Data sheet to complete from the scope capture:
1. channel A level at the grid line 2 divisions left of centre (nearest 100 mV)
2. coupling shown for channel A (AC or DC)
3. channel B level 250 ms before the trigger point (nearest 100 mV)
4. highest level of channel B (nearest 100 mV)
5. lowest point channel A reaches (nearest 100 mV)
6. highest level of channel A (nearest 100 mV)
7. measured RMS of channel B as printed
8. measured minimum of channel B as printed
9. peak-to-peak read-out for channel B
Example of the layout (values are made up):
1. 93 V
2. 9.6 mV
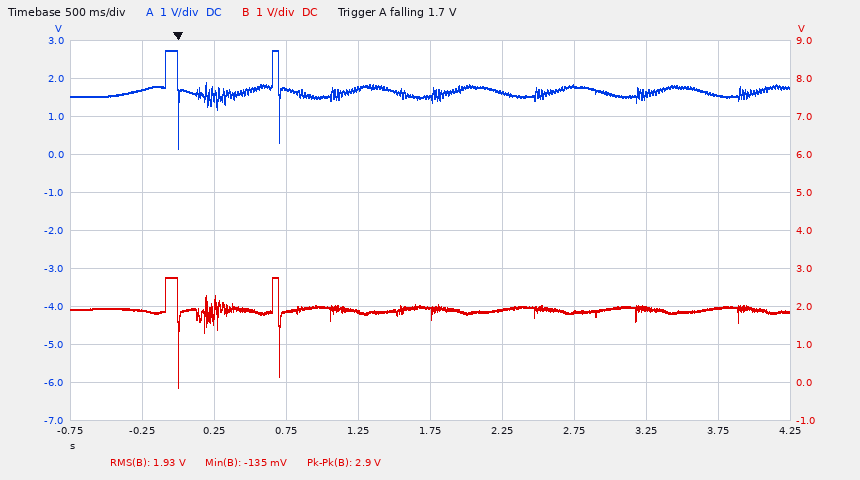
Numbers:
1. 1.7 V
2. DC
3. 1.9 V
4. 2.8 V
5. 200 mV
6. 2.7 V
7. 1.93 V
8. -135 mV
9. 2.9 V
